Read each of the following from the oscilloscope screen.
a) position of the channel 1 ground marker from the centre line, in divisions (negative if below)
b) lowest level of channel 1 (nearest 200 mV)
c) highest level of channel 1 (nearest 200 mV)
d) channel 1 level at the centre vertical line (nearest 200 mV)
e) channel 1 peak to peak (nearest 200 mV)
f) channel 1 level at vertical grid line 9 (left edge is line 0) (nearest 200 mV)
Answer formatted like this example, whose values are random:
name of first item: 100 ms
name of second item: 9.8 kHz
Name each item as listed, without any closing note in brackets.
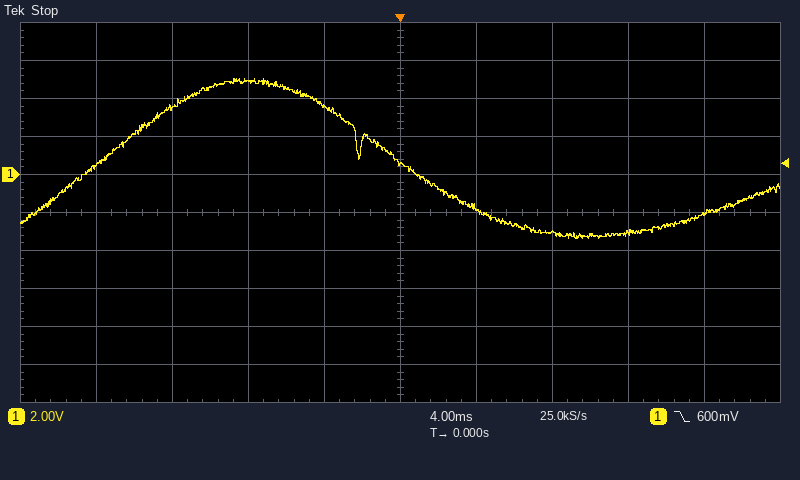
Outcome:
position of the channel 1 ground marker from the centre line, in divisions: +1.0 div
lowest level of channel 1: -3.4 V
highest level of channel 1: 5.0 V
channel 1 level at the centre vertical line: 600 mV
channel 1 peak to peak: 8.4 V
channel 1 level at vertical grid line 9 (left edge is line 0): -2.0 V
